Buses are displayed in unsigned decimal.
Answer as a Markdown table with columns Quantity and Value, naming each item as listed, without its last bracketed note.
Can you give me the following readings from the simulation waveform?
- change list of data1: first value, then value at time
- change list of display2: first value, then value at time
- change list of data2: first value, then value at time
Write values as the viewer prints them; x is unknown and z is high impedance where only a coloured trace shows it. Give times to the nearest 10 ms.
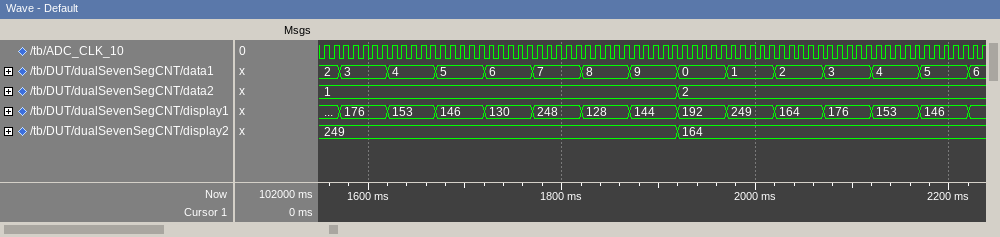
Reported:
| Quantity | Value |
|---|---|
| change list of data1: first value, then value at time | 2, 3 at 1570 ms, 4 at 1620 ms, 5 at 1670 ms, 6 at 1720 ms, 7 at 1770 ms, 8 at 1820 ms, 9 at 1870 ms, 0 at 1920 ms, 1 at 1970 ms, 2 at 2020 ms, 3 at 2070 ms, 4 at 2120 ms, 5 at 2170 ms, 6 at 2220 ms |
| change list of display2: first value, then value at time | 249, 164 at 1920 ms |
| change list of data2: first value, then value at time | 1, 2 at 1920 ms |
